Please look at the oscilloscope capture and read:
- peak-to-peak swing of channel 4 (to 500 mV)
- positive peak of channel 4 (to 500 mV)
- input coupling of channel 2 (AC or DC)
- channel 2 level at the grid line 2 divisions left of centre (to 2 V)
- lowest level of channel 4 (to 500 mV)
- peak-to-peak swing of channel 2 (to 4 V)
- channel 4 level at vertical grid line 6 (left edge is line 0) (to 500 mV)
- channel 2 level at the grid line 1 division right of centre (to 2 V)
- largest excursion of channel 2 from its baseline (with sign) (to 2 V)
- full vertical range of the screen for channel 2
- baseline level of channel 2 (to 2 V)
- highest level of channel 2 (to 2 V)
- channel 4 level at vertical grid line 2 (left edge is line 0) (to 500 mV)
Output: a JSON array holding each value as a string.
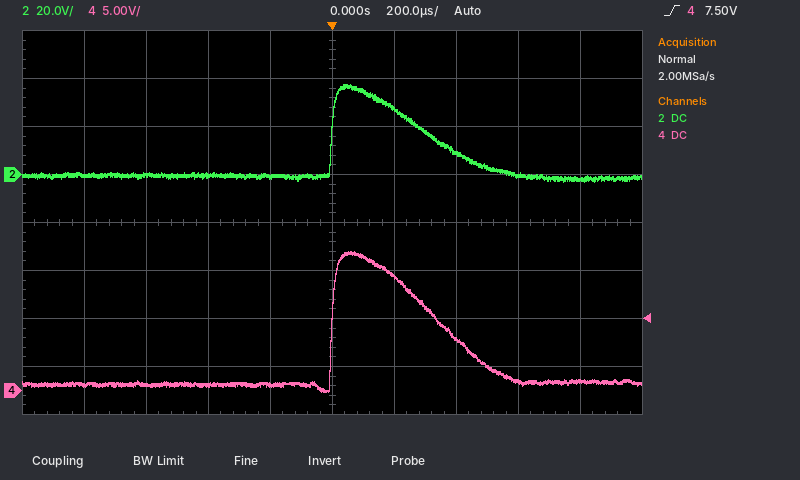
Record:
["14.5 V", "14.5 V", "DC", "0 V", "0.0 V", "40 V", "12.0 V", "28 V", "+38 V", "160 V", "0 V", "38 V", "500 mV"]
